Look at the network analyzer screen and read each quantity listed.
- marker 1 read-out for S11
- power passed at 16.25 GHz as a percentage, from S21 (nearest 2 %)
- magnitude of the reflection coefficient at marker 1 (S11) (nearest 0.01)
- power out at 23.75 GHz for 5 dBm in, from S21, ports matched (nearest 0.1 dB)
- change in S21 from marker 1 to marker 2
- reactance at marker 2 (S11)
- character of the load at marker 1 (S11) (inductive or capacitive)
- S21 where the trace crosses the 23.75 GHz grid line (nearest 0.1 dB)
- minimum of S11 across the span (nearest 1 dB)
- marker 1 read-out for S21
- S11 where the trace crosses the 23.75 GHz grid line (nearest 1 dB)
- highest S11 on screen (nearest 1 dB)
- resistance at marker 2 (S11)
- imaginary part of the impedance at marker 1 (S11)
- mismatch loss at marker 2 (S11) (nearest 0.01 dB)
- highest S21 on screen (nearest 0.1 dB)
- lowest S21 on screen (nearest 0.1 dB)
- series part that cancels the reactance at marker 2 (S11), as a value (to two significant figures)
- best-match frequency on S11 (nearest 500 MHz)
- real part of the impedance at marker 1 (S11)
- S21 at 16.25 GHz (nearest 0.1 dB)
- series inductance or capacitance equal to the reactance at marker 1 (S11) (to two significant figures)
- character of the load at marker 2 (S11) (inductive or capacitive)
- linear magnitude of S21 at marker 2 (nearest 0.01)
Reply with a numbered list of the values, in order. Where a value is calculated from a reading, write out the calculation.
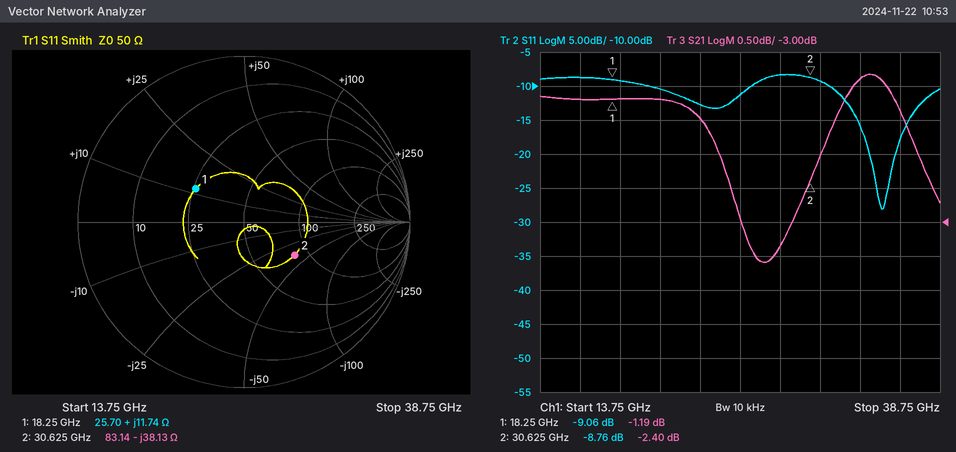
1. -9.06 dB
2. 10^(-1.2/10) ≈ 76 %
3. 0.35
4. 5 dBm + (-1.5 dB) = 3.5 dBm
5. -2.4 − (-1.19) = -1.21 dB
6. -38.13 Ω
7. inductive
8. -1.5 dB
9. -28 dB
10. -1.19 dB
11. -13 dB
12. -8 dB
13. 83.14 Ω
14. +11.74 Ω
15. −10 log10(1 − 10^(-8.76/10)) ≈ 0.62 dB
16. -0.8 dB
17. -3.6 dB
18. L = 38.13 Ω/(2π × 30.625 GHz) ≈ 198 pH, so 200 pH to two significant figures
19. 35.0 GHz
20. 25.70 Ω
21. -1.2 dB
22. L = 11.74 Ω/(2π × 18.25 GHz) ≈ 102 pH, so 100 pH to two significant figures
23. capacitive
24. 10^(-2.4/20) ≈ 0.76
